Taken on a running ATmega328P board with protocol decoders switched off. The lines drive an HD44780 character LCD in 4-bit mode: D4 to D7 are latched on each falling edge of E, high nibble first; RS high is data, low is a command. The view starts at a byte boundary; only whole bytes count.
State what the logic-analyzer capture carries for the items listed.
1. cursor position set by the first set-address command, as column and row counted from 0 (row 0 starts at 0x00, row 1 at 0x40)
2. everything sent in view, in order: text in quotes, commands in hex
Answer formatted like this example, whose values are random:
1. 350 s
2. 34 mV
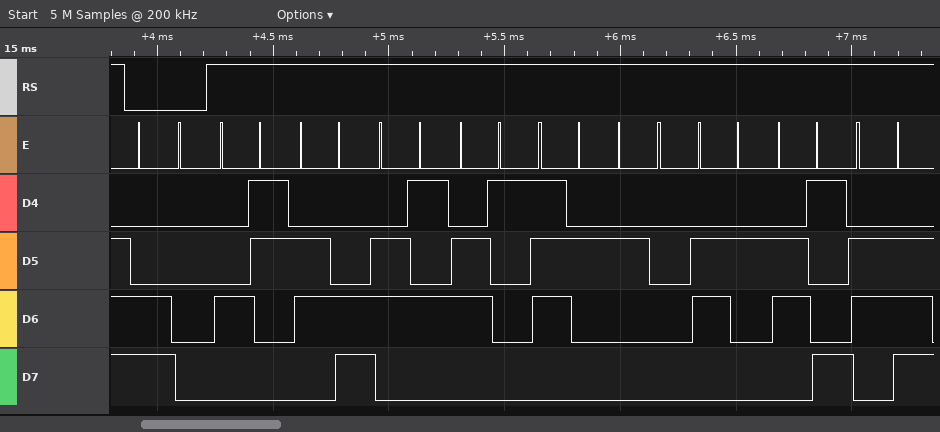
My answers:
1. column 0, row 1
2. 0xC0 "Clear bin"
